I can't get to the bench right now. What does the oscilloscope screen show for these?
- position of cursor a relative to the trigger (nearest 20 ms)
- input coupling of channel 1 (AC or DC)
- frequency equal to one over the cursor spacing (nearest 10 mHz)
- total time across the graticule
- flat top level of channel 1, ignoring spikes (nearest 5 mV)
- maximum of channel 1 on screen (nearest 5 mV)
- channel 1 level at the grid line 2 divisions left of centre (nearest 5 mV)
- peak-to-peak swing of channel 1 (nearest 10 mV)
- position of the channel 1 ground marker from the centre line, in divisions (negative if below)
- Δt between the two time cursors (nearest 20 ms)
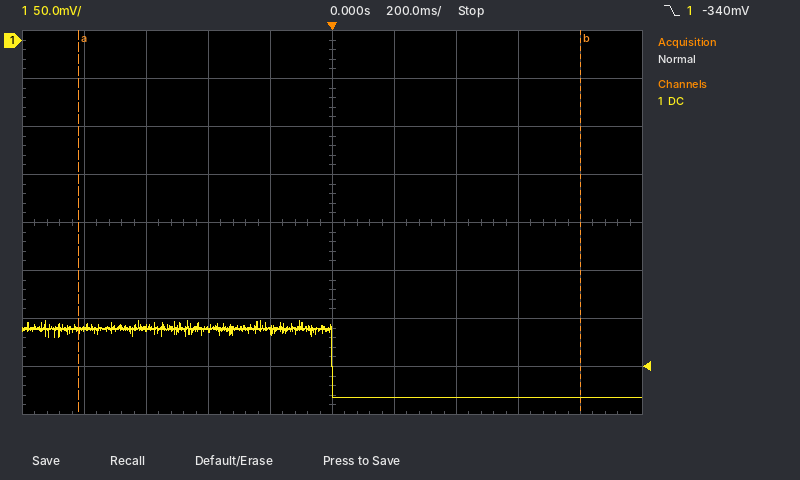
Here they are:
-820 ms
DC
620 mHz
2 s
-300 mV
-290 mV
-300 mV
80 mV
+3.8 div
1.62 s
